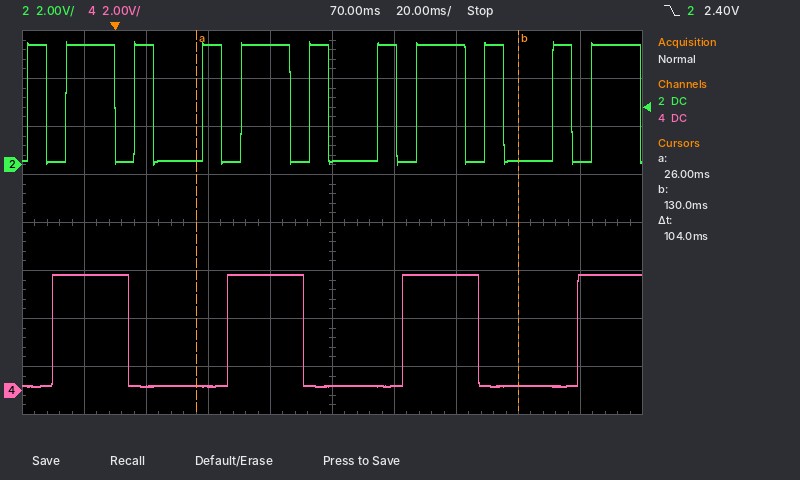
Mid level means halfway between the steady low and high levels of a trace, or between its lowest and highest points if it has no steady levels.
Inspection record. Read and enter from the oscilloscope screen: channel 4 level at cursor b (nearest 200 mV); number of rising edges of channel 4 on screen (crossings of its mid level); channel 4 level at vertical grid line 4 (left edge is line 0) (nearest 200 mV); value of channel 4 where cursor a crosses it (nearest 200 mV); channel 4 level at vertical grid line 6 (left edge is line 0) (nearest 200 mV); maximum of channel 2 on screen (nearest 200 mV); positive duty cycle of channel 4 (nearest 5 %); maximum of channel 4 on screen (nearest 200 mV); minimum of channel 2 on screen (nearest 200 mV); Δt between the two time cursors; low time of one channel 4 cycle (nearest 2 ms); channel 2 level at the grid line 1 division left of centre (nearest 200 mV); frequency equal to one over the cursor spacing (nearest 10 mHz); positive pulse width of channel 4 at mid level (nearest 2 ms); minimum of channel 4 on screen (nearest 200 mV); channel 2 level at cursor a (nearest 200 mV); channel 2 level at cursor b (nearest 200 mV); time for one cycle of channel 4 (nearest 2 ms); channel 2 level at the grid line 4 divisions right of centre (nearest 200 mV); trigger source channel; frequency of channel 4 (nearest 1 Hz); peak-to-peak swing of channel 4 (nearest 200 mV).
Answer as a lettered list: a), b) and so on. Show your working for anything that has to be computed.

a) 200 mV
b) 4
c) 4.8 V
d) 200 mV
e) 200 mV
f) 5.2 V
g) 24 ms / 56 ms ≈ 42.9 %, so 45 % to the nearest 5 %
h) 4.8 V
i) 0.0 V
j) 104 ms
k) 32 ms
l) 5.0 V
m) 1 / 104 ms ≈ 9.62 Hz
n) 24 ms
o) 200 mV
p) 200 mV
q) 200 mV
r) 56 ms
s) 200 mV
t) channel 2
u) 1 / 56 ms ≈ 18 Hz
v) 4.8 V − (200 mV) = 4.6 V
